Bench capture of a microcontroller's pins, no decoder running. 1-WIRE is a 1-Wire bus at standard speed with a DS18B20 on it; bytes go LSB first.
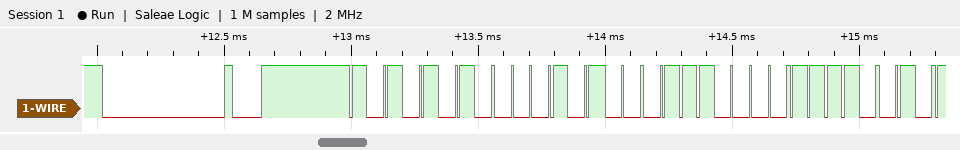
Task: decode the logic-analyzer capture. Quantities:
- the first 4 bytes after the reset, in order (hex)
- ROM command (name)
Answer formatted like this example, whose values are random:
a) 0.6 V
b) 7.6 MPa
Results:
a) 55 28 0E 4F
b) Match ROM
